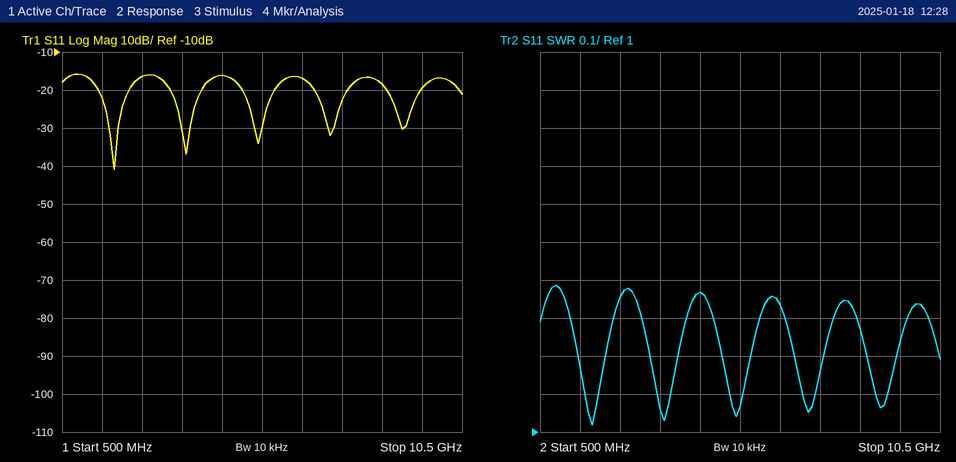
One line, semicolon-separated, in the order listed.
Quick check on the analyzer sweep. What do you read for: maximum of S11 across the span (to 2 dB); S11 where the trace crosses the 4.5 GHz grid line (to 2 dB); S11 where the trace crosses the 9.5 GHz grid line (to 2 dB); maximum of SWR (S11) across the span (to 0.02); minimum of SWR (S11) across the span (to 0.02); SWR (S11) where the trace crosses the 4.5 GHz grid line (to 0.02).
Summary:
-16 dB; -16 dB; -20 dB; 1.38; 1.02; 1.36
